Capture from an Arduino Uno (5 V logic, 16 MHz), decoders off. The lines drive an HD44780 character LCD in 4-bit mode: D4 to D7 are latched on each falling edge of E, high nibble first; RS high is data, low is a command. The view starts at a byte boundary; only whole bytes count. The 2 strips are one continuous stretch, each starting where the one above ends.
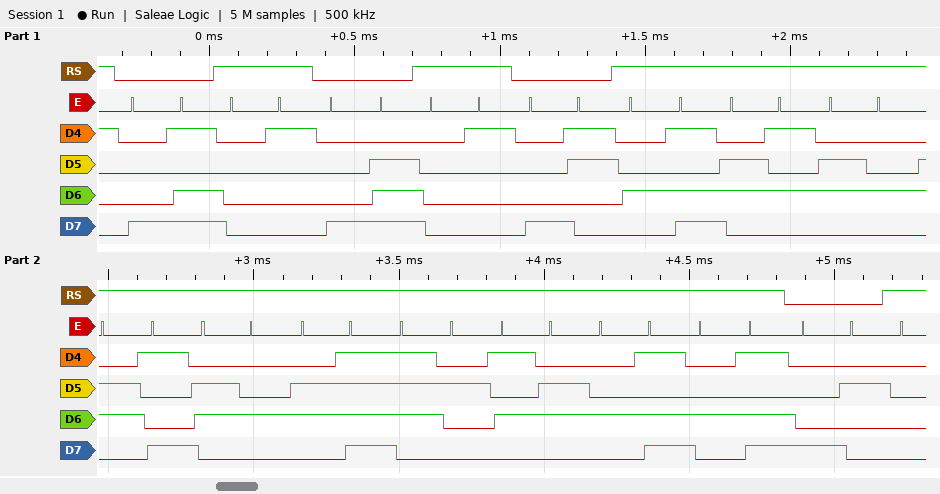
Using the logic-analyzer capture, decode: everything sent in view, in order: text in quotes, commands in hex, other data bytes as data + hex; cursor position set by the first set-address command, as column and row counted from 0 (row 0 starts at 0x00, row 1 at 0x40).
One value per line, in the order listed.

0x8D data 01 0x8E data 01 0x83 "MedidorVMM" 0x82
column 13, row 0
